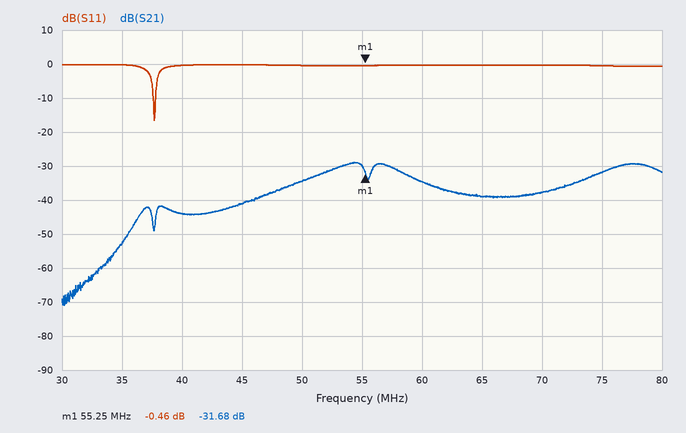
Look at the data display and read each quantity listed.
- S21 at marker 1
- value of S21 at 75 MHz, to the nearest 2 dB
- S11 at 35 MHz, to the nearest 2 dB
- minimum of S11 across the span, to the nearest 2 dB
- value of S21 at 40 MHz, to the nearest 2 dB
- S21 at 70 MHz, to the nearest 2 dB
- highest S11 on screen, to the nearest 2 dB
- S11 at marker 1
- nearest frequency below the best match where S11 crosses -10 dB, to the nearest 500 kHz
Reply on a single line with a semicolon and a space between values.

-31.68 dB; -32 dB; 0 dB; -16 dB; -44 dB; -38 dB; 0 dB; -0.46 dB; 37.5 MHz
